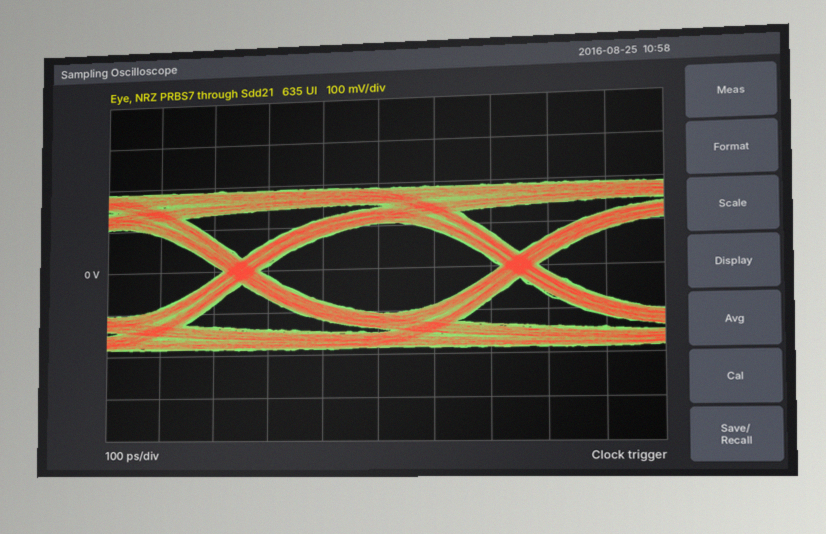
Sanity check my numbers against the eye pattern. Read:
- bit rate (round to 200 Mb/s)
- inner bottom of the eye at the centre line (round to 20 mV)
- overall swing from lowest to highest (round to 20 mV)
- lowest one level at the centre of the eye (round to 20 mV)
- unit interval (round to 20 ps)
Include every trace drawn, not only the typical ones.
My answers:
2.0 Gb/s
-100 mV
380 mV
100 mV
500 ps
